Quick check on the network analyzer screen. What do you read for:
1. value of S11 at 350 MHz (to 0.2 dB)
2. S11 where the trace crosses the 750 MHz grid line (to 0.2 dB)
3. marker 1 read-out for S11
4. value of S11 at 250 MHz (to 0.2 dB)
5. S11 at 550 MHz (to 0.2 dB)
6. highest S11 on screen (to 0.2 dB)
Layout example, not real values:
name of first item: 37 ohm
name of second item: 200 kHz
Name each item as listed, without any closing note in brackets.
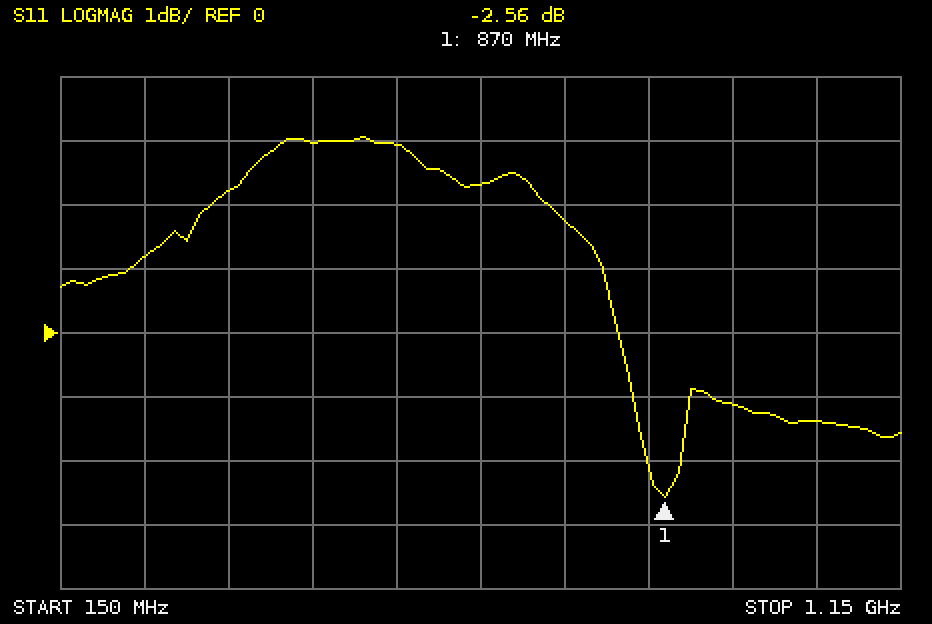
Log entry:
value of S11 at 350 MHz: 2.2 dB
S11 where the trace crosses the 750 MHz grid line: 1.8 dB
marker 1 read-out for S11: -2.56 dB
value of S11 at 250 MHz: 1.2 dB
S11 at 550 MHz: 3.0 dB
highest S11 on screen: 3.0 dB
